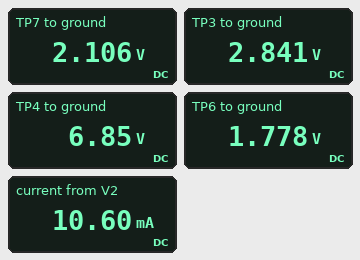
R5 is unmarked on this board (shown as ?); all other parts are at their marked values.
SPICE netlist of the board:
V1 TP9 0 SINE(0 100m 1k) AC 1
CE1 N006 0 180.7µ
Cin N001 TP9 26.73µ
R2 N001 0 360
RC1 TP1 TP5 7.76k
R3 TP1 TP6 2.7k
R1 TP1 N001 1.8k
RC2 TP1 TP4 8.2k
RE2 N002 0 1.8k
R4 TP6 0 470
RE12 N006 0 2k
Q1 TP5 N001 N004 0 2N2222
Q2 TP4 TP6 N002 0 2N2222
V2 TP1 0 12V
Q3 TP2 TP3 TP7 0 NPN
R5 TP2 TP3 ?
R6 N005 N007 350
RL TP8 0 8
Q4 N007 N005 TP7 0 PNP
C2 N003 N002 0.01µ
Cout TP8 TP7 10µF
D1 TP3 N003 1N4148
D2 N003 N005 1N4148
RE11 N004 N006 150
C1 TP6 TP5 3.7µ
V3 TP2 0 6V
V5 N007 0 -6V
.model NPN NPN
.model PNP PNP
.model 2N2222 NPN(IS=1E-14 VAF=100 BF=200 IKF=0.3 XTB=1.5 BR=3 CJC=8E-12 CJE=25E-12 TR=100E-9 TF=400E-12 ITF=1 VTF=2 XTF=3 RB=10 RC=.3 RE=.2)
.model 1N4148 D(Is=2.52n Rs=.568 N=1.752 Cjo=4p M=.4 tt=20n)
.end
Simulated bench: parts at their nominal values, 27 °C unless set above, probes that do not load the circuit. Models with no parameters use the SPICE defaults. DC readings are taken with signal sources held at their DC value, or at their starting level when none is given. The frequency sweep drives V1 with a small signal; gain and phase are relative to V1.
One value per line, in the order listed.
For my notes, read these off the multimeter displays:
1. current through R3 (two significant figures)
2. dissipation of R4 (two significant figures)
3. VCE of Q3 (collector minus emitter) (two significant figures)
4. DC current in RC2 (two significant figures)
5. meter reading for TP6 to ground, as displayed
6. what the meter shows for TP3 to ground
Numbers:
3.8 mA
6.7 mW
3.9 V
630 µA
1.778 V
2.841 V
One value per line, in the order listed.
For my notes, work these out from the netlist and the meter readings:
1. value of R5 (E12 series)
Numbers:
150 Ω
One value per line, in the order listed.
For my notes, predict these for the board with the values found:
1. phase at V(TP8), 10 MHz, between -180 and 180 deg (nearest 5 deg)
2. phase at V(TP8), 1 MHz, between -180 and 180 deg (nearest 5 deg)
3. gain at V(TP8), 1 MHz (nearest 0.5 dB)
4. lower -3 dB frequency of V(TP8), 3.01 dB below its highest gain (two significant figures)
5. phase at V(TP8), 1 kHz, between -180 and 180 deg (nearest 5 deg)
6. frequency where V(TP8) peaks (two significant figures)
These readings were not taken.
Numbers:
150 deg
155 deg
-18.0 dB
97 kHz
-75 deg
370 kHz
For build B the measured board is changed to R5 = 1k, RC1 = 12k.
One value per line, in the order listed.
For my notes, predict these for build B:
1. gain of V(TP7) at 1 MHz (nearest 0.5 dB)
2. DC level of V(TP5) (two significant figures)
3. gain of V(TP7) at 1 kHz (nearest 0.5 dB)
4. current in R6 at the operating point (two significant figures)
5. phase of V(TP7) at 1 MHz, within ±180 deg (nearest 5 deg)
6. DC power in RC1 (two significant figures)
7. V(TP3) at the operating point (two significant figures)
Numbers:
-31.5 dB
4.5 V
-58.0 dB
7.9 mA
165 deg
4.7 mW
-1.9 V
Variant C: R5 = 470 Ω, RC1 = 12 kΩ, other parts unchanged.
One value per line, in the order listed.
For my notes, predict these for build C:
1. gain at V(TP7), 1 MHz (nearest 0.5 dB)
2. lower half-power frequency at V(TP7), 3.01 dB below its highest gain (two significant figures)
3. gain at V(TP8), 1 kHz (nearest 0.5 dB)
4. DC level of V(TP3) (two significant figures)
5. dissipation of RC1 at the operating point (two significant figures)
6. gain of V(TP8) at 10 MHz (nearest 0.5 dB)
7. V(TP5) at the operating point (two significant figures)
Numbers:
-24.0 dB
62 kHz
-59.0 dB
-67 mV
4.7 mW
-31.5 dB
4.5 V
